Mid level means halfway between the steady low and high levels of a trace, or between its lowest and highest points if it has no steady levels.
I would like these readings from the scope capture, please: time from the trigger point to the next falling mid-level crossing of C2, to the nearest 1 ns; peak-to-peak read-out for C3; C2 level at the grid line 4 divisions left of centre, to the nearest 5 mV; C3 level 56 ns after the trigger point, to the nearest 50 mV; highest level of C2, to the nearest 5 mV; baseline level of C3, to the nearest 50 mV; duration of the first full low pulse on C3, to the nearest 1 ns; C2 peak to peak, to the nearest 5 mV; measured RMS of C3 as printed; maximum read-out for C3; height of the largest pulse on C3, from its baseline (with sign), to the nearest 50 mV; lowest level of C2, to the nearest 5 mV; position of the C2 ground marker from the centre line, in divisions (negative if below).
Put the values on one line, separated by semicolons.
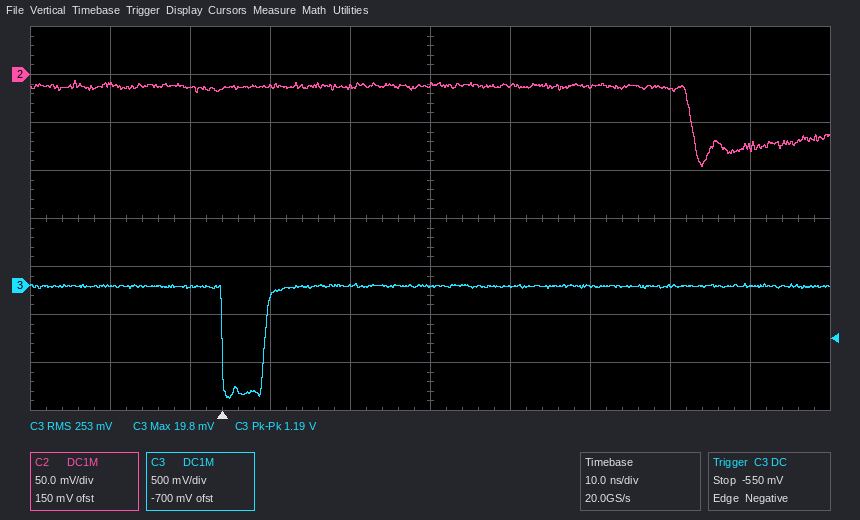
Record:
59 ns; 1.19 V; -10 mV; 0 mV; -5 mV; 0 mV; 5 ns; 90 mV; 253 mV; 19.8 mV; -1.15 V; -95 mV; +3.0 div
